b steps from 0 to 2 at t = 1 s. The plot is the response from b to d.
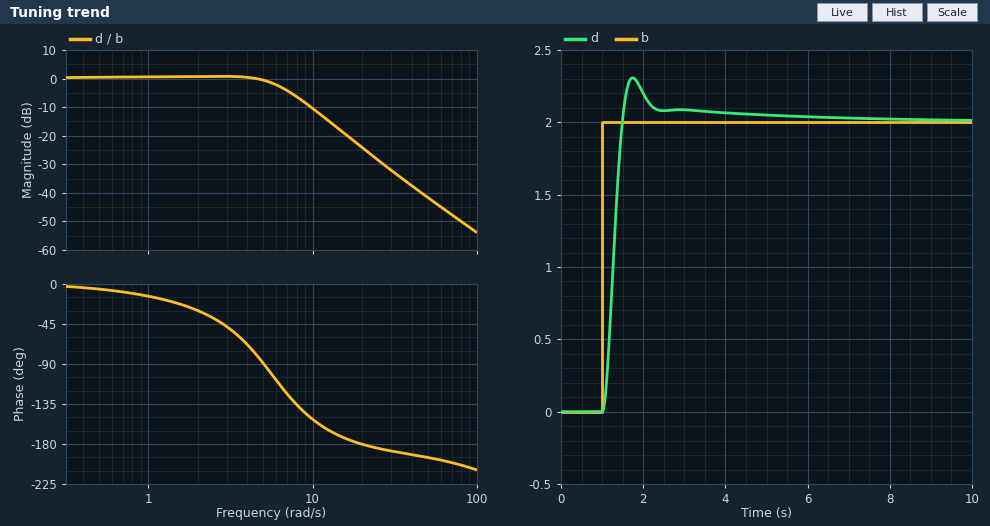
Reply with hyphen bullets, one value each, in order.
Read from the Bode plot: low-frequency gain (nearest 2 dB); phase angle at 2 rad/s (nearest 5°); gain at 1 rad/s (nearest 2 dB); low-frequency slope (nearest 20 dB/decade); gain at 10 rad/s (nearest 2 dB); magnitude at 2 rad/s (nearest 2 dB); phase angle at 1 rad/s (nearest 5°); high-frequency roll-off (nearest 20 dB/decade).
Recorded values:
- 0 dB
- -30°
- 0 dB
- 0 dB/decade
- -10 dB
- 0 dB
- -15°
- -40 dB/decade
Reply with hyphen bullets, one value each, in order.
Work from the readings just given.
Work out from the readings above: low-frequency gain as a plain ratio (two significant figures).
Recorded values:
- 1.0
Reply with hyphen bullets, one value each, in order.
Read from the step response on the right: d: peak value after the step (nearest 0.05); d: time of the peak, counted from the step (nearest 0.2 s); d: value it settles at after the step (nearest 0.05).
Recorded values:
- 2.30
- 0.8 s
- 2.00
